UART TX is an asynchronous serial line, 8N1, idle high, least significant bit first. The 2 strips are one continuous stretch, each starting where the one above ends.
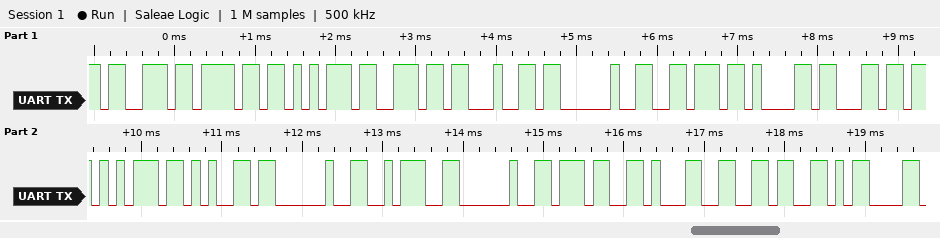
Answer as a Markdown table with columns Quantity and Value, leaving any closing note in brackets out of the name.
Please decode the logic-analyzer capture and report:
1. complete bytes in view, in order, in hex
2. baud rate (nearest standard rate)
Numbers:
| Quantity | Value |
|---|---|
| complete bytes in view, in order, in hex | 73 6F 75 6E 64 20 76 61 6C 75 65 20 3A 20 37 31 36 0D |
| baud rate | 9600 baud |
